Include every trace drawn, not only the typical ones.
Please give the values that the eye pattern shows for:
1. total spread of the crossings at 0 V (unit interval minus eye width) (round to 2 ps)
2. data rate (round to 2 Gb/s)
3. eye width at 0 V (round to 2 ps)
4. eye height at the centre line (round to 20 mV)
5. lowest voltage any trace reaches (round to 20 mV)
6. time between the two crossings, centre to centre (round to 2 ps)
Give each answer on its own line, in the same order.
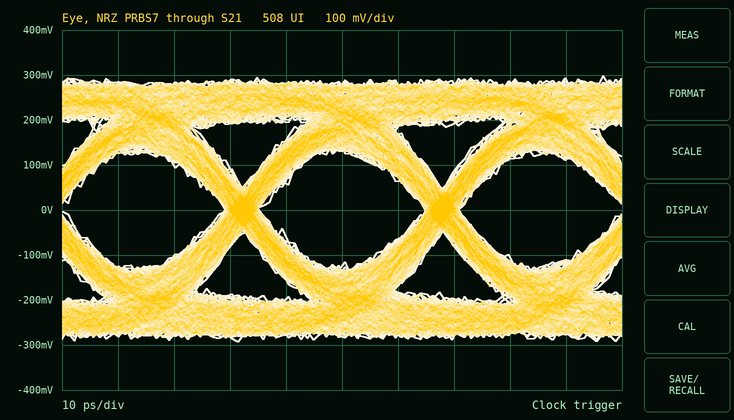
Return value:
6 ps
28 Gb/s
30 ps
260 mV
-300 mV
36 ps
